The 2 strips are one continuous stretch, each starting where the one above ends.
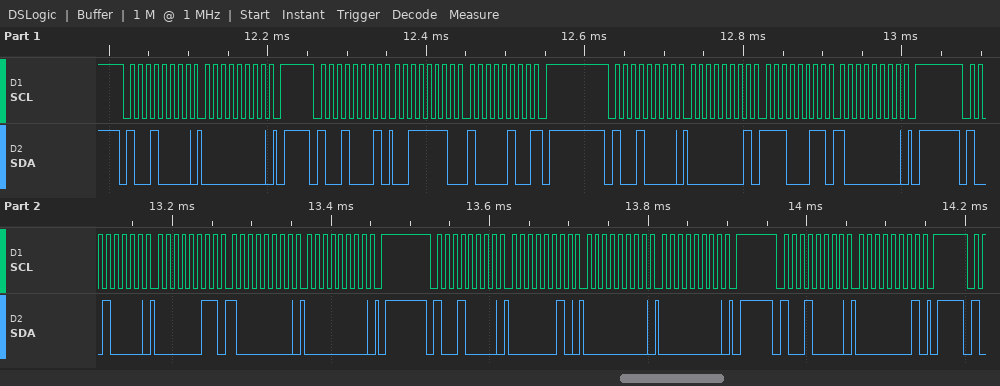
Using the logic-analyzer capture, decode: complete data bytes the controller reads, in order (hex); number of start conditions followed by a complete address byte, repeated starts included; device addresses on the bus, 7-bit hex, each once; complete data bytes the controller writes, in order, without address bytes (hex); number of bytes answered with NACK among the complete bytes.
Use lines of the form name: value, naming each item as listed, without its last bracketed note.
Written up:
complete data bytes the controller reads, in order: 3E 84
number of start conditions followed by a complete address byte, repeated starts included: 6
device addresses on the bus, 7-bit hex, each once: 0x48
complete data bytes the controller writes, in order, without address bytes: 00 01 E3 80 03 80 00 02 00 00 01
number of bytes answered with NACK among the complete bytes: 1
